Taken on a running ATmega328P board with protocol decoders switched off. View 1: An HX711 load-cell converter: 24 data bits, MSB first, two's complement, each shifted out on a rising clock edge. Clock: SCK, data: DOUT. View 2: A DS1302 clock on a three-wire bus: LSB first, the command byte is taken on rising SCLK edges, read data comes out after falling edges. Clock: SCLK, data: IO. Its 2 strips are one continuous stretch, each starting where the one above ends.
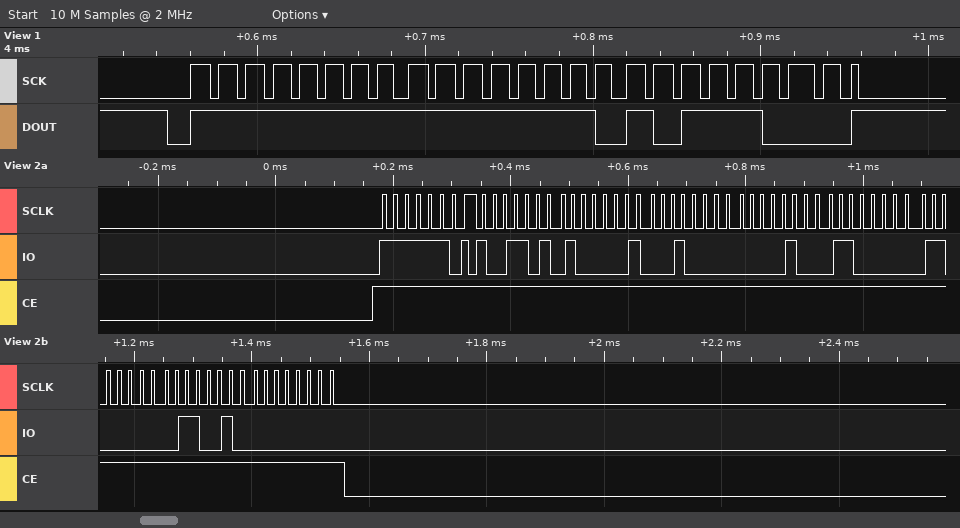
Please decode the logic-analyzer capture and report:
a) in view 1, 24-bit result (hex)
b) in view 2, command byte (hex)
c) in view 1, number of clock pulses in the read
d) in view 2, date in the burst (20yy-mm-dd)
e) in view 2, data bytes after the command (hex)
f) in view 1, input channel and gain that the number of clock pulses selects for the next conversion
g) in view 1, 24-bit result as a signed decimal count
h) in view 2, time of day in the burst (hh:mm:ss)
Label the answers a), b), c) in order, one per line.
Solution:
a) 0xFFFEB8
b) 0xBF
c) 25
d) 2026-03-10
e) 59 41 04 10 03 03 26 00
f) channel A, gain 128
g) -328
h) 04:41:59
